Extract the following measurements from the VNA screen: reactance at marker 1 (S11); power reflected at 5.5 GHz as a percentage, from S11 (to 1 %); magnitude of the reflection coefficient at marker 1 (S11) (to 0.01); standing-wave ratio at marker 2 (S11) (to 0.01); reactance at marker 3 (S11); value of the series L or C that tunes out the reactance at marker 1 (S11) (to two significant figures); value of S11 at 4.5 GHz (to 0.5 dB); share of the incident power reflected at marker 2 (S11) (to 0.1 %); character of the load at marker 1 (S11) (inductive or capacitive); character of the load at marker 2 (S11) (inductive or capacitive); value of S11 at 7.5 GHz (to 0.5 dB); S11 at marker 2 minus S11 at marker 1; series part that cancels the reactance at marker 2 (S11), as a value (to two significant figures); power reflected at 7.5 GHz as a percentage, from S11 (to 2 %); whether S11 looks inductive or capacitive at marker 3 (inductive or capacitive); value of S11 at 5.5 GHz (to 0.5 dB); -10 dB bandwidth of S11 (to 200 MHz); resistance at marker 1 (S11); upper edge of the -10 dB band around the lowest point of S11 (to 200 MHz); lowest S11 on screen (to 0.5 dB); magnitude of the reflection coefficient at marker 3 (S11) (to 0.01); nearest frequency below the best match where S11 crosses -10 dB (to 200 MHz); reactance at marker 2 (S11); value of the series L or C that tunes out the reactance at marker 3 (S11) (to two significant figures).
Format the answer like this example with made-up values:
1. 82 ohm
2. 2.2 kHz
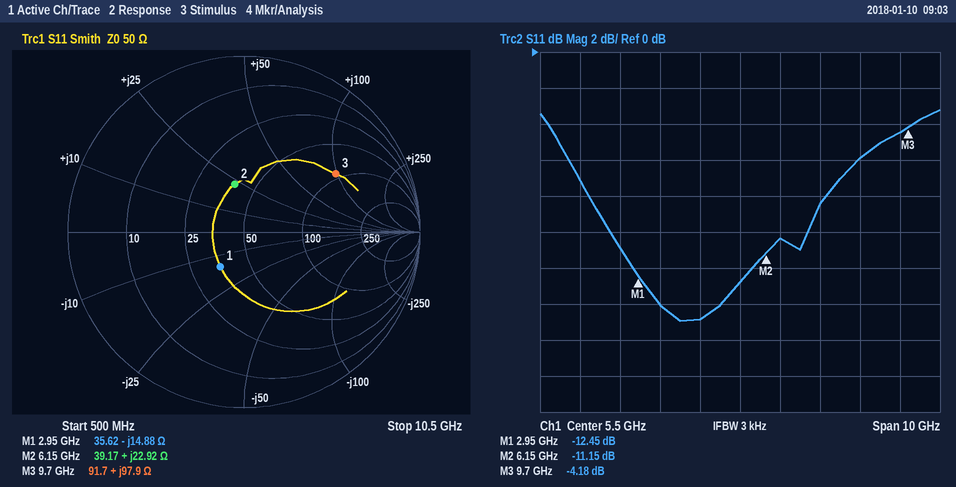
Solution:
1. -14.88 Ω
2. 5 %
3. 0.24
4. 1.76
5. +97.9 Ω
6. 800 pH
7. -15.0 dB
8. 7.7 %
9. capacitive
10. inductive
11. -8.5 dB
12. 1.30 dB
13. 1.1 pF
14. 14 %
15. inductive
16. -13.0 dB
17. 5.0 GHz
18. 35.62 Ω
19. 7.2 GHz
20. -15.0 dB
21. 0.62
22. 2.2 GHz
23. +22.92 Ω
24. 170 fF
